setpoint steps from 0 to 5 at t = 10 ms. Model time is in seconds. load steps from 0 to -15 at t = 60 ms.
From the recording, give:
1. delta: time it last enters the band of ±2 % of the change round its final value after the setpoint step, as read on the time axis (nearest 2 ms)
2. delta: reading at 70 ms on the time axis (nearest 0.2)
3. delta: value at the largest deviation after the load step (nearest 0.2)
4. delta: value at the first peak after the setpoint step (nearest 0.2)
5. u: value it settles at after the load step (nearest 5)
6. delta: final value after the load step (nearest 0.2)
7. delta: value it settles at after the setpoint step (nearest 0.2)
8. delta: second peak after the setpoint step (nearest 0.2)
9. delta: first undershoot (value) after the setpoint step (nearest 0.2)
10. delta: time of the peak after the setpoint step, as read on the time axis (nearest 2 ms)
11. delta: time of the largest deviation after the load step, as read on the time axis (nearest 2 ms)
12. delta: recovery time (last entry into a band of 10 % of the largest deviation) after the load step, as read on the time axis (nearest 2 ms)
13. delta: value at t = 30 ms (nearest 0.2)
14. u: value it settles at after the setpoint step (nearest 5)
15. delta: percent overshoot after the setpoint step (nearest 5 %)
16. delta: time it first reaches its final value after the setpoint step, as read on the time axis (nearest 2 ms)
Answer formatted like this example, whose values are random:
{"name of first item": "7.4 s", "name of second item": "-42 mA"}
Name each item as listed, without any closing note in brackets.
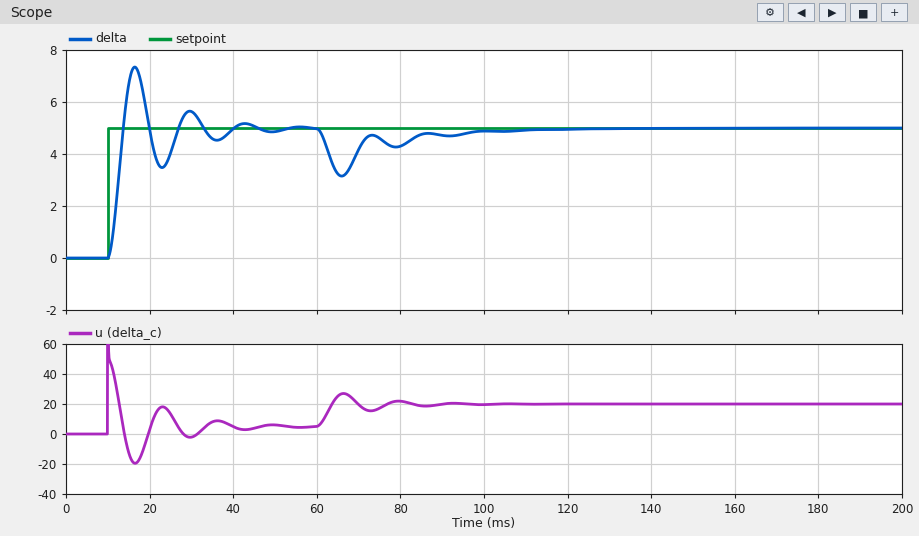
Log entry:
{"delta: time it last enters the band of ±2 % of the change round its final value after the setpoint step, as read on the time axis": "52 ms", "delta: reading at 70 ms on the time axis": "4.2", "delta: value at the largest deviation after the load step": "3.2", "delta: value at the first peak after the setpoint step": "7.4", "u: value it settles at after the load step": "20", "delta: final value after the load step": "5.0", "delta: value it settles at after the setpoint step": "5.0", "delta: second peak after the setpoint step": "5.6", "delta: first undershoot (value) after the setpoint step": "3.4", "delta: time of the peak after the setpoint step, as read on the time axis": "16 ms", "delta: time of the largest deviation after the load step, as read on the time axis": "66 ms", "delta: recovery time (last entry into a band of 10 % of the largest deviation) after the load step, as read on the time axis": "96 ms", "delta: value at t = 30 ms": "5.6", "u: value it settles at after the setpoint step": "5", "delta: percent overshoot after the setpoint step": "45 %", "delta: time it first reaches its final value after the setpoint step, as read on the time axis": "14 ms"}
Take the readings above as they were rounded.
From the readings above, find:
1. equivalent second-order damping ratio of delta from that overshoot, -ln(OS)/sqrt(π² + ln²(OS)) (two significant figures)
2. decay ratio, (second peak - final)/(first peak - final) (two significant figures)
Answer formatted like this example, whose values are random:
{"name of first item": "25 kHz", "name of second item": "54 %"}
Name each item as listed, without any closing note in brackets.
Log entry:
{"equivalent second-order damping ratio of delta from that overshoot, -ln(OS)/sqrt(π² + ln²(OS))": "0.25", "decay ratio, (second peak - final)/(first peak - final)": "0.25"}
